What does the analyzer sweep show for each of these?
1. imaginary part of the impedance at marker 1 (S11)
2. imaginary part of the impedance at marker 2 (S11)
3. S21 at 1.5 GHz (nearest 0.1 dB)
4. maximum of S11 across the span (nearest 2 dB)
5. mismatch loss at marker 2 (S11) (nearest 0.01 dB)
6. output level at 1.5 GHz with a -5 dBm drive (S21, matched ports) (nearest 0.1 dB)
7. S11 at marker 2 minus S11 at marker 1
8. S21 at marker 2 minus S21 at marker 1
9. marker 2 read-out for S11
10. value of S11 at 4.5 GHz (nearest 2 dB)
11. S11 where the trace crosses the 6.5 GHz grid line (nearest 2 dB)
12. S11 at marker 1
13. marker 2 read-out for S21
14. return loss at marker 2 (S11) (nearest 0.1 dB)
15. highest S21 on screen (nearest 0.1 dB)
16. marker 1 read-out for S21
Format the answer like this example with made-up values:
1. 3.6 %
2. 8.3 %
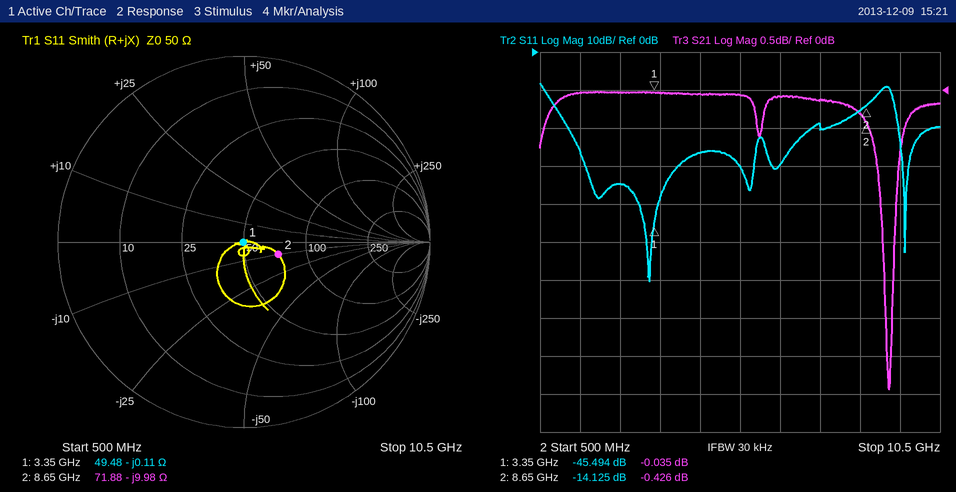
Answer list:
1. -0.11 Ω
2. -9.98 Ω
3. 0.0 dB
4. -8 dB
5. 0.17 dB
6. -5.0 dBm
7. 31.369 dB
8. -0.391 dB
9. -14.125 dB
10. -26 dB
11. -30 dB
12. -45.494 dB
13. -0.426 dB
14. 14.1 dB
15. 0.0 dB
16. -0.035 dB
